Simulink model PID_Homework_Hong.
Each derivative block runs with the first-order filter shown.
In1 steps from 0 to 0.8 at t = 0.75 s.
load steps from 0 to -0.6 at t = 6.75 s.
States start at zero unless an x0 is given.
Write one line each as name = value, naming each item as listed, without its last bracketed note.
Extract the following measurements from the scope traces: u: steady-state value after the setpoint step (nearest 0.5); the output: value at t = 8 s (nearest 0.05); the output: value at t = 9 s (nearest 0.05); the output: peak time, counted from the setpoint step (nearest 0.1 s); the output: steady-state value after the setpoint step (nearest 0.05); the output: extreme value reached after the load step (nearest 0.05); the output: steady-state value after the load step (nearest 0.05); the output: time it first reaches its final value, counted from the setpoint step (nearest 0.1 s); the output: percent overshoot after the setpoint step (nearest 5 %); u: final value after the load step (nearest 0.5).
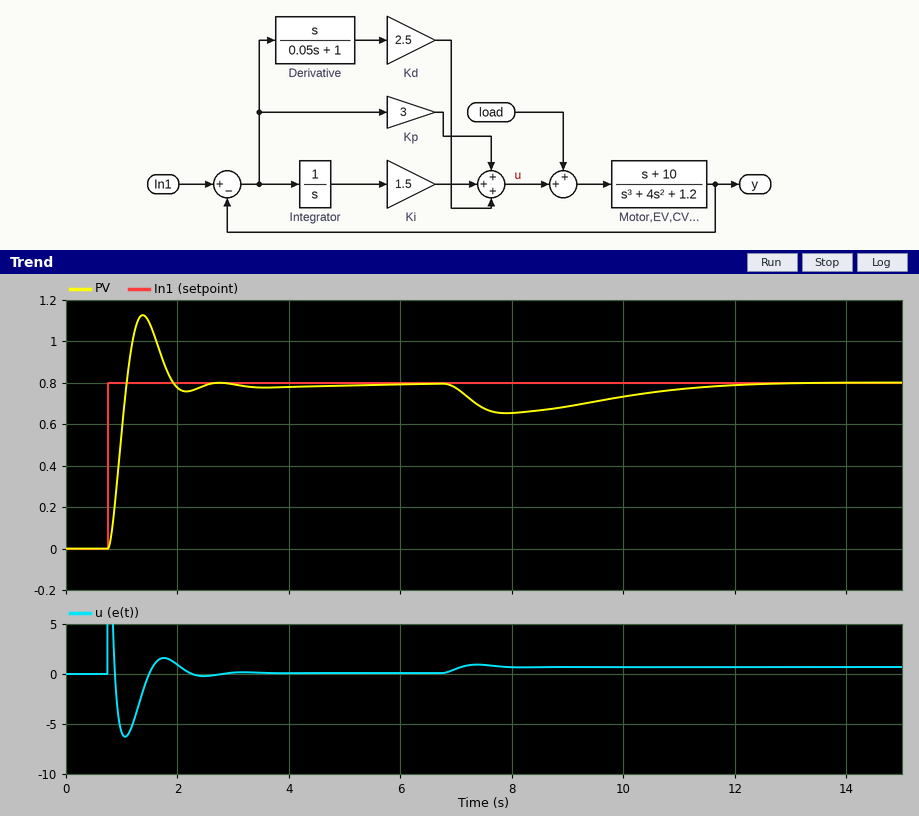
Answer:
u: steady-state value after the setpoint step = 0.0
the output: value at t = 8 s = 0.65
the output: value at t = 9 s = 0.70
the output: peak time, counted from the setpoint step = 0.6 s
the output: steady-state value after the setpoint step = 0.80
the output: extreme value reached after the load step = 0.65
the output: steady-state value after the load step = 0.80
the output: time it first reaches its final value, counted from the setpoint step = 0.3 s
the output: percent overshoot after the setpoint step = 40 %
u: final value after the load step = 0.5
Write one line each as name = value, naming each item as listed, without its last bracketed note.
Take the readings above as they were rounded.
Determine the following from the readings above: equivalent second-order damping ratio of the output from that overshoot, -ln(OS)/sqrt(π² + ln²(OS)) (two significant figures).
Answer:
equivalent second-order damping ratio of the output from that overshoot, -ln(OS)/sqrt(π² + ln²(OS)) = 0.28
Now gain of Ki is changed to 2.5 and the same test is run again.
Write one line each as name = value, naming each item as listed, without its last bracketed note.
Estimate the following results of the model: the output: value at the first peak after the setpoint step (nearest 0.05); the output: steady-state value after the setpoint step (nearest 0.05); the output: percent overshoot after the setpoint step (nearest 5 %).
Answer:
the output: value at the first peak after the setpoint step = 1.15
the output: steady-state value after the setpoint step = 0.80
the output: percent overshoot after the setpoint step = 45 %
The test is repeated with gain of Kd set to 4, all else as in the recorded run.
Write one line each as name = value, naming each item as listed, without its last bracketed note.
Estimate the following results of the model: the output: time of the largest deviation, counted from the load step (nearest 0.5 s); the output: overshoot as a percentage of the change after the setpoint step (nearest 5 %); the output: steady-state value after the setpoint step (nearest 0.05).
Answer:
the output: time of the largest deviation, counted from the load step = 2.0 s
the output: overshoot as a percentage of the change after the setpoint step = 35 %
the output: steady-state value after the setpoint step = 0.80
